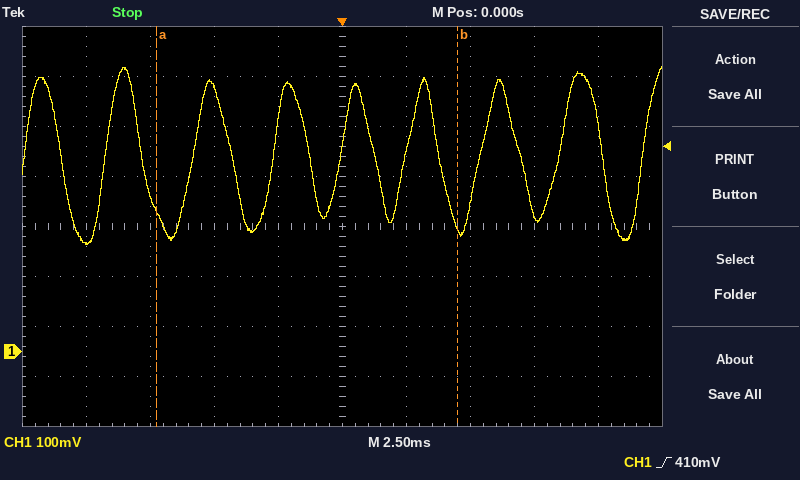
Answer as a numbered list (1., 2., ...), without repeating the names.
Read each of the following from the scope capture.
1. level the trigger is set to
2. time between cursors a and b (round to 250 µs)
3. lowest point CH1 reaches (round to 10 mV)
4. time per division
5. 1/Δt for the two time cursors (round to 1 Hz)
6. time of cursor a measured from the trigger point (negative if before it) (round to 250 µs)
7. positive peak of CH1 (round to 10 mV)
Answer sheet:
1. 410 mV
2. 11.75 ms
3. 210 mV
4. 2.5 ms
5. 85 Hz
6. -7.25 ms
7. 570 mV
